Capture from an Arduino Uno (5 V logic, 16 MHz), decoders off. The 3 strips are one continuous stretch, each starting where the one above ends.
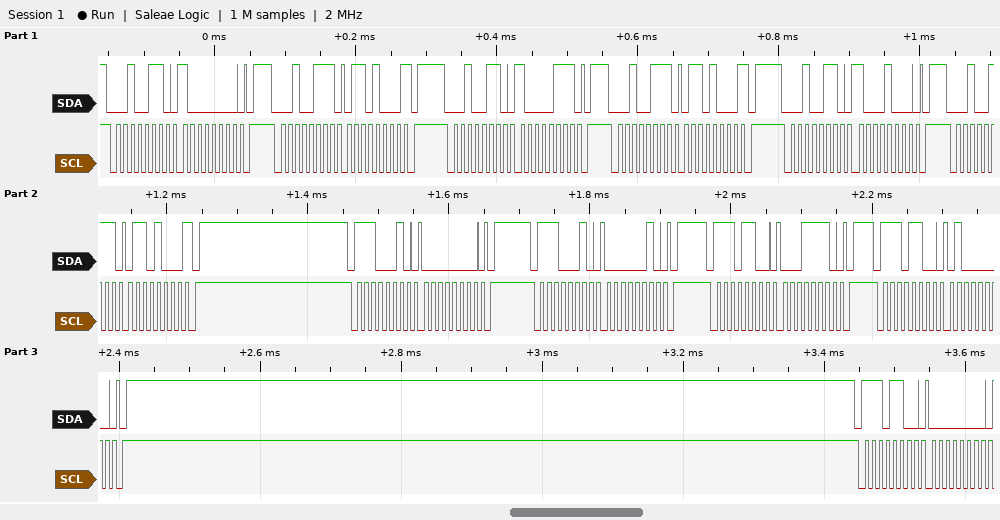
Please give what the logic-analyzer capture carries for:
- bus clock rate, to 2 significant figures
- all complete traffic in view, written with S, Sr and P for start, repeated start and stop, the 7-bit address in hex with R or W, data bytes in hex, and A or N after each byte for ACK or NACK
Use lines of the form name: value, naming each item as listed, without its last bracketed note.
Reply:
bus clock rate, to 2 significant figures: 100 kHz
all complete traffic in view, written with S, Sr and P for start, repeated start and stop, the 7-bit address in hex with R or W, data bytes in hex, and A or N after each byte for ACK or NACK: S 13W A 80 A P S 13R A 68 N P S 13W A 87 A P S 13R A 68 N P S 13W A 88 A P S 13R A 68 N P S 71W A 00 A P S 71W A 02 A P S 76W A 1E A P S 76W A 40 A P S 76W A 00 A
